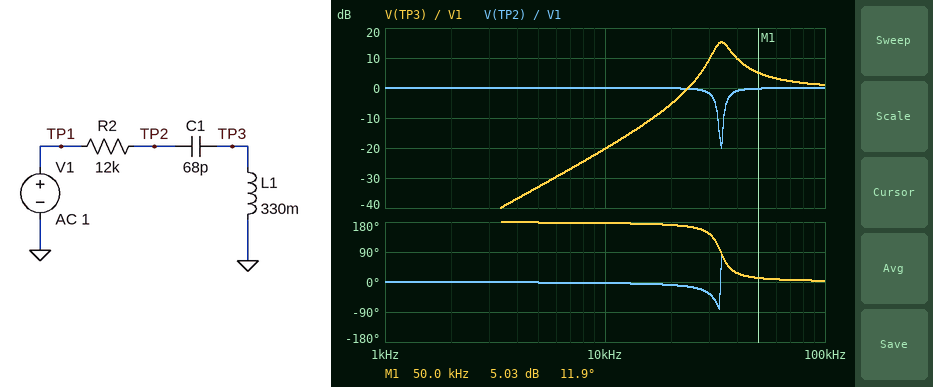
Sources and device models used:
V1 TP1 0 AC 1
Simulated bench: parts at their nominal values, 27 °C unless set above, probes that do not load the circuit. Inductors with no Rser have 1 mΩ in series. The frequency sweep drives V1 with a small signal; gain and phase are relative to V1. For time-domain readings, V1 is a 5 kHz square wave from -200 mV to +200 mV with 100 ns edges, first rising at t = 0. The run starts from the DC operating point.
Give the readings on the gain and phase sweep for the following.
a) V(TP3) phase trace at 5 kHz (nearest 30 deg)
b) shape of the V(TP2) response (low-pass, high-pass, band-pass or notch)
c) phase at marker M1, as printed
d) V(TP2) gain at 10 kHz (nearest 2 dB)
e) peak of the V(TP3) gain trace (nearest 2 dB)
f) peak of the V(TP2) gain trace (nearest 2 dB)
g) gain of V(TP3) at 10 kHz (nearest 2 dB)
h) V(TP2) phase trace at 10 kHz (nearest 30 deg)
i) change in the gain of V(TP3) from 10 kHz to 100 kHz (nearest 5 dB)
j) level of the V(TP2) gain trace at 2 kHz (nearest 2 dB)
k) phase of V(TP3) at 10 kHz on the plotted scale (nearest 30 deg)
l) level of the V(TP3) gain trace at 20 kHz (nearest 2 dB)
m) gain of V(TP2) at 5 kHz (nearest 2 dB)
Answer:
180 deg
notch
11.9 deg
0 dB
16 dB
0 dB
-20 dB
0 deg
20 dB
0 dB
180 deg
-6 dB
0 dB
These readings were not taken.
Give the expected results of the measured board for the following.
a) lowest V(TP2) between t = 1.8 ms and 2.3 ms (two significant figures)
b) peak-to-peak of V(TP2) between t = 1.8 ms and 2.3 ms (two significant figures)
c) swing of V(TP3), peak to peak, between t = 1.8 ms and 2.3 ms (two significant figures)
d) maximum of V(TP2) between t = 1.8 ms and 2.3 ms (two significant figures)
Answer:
-250 mV
500 mV
870 mV
250 mV
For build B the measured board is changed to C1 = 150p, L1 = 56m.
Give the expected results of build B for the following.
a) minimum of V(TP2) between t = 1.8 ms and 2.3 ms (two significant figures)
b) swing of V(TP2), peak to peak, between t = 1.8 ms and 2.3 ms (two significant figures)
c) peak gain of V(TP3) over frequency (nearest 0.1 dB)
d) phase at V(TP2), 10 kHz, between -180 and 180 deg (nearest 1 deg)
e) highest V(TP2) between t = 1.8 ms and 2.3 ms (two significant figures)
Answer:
-260 mV
520 mV
4.6 dB
-7 deg
260 mV
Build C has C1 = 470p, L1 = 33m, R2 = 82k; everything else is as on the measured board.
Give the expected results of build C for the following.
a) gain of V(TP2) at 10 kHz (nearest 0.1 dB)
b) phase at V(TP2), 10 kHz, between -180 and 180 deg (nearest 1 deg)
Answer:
-8.8 dB
-69 deg
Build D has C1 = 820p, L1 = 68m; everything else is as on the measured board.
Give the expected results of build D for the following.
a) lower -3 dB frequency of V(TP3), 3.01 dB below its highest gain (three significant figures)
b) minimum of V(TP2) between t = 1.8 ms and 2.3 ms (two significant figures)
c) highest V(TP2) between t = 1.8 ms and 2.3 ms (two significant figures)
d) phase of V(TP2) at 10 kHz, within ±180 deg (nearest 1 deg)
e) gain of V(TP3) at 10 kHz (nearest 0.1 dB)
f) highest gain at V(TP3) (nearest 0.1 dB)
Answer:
20.1 kHz
-220 mV
220 mV
-38 deg
-13.1 dB
0.1 dB
